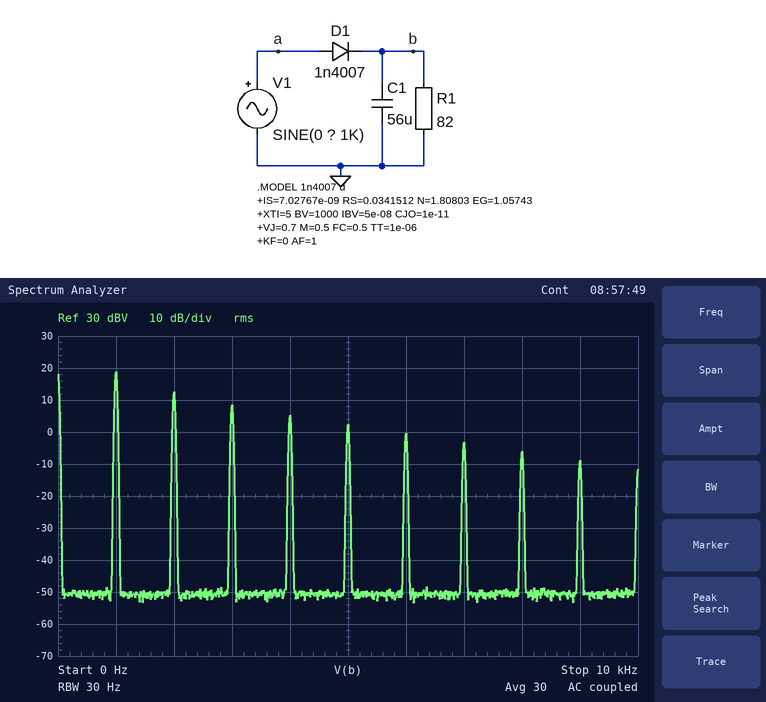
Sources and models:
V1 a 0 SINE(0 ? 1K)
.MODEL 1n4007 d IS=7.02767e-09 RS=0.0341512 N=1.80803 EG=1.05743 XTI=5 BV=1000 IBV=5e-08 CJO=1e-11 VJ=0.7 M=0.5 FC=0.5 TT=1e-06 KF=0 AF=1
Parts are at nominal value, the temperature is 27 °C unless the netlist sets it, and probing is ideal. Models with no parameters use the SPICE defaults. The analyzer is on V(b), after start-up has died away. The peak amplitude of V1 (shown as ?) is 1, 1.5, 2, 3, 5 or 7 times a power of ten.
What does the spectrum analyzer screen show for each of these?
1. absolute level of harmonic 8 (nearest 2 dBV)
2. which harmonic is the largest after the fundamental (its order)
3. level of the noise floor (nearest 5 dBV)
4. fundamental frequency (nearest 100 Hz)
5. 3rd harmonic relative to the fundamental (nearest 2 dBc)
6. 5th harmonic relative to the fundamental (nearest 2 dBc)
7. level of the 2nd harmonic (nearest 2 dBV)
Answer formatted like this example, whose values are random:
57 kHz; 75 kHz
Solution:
-6 dBV; 2; -50 dBV; 1.0 kHz; -10 dBc; -16 dBc; 12 dBV
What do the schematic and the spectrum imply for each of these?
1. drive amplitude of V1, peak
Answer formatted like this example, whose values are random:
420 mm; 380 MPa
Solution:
200 V
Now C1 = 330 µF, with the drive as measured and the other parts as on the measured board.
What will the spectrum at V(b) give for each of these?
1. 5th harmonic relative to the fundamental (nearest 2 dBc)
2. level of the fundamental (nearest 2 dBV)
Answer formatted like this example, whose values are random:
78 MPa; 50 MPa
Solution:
-14 dBc; 4 dBV
